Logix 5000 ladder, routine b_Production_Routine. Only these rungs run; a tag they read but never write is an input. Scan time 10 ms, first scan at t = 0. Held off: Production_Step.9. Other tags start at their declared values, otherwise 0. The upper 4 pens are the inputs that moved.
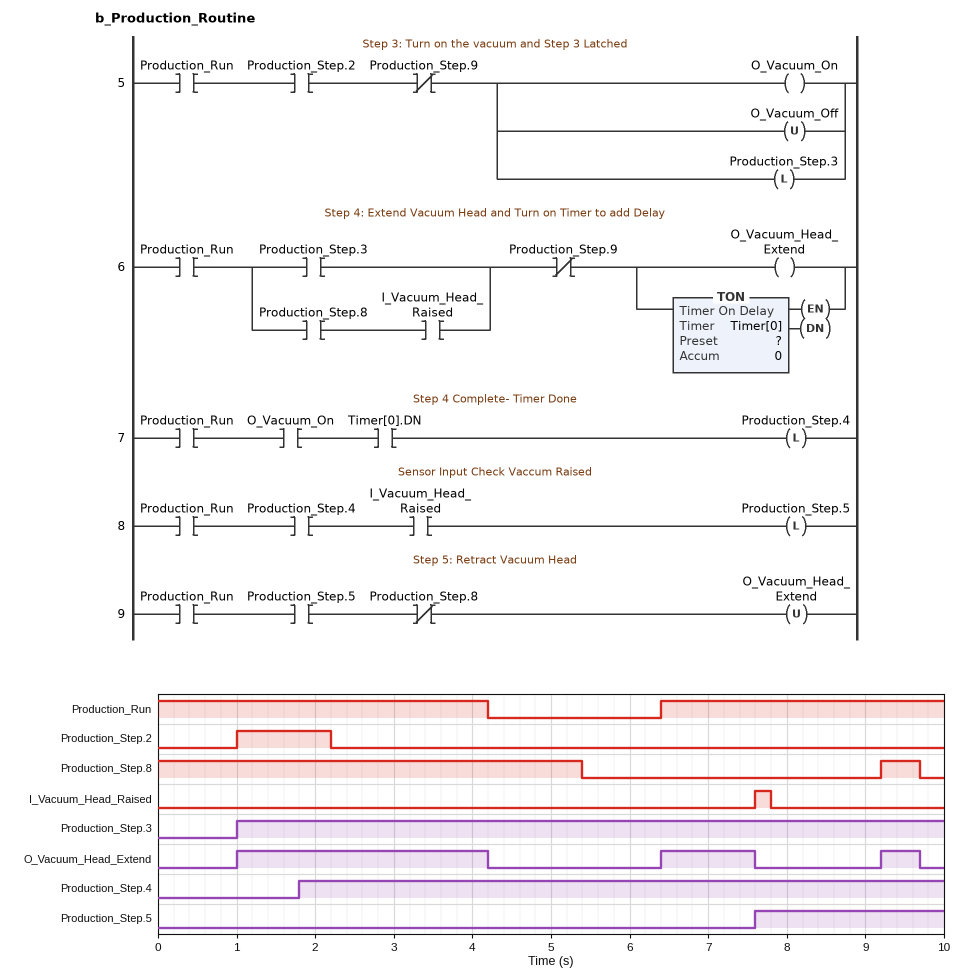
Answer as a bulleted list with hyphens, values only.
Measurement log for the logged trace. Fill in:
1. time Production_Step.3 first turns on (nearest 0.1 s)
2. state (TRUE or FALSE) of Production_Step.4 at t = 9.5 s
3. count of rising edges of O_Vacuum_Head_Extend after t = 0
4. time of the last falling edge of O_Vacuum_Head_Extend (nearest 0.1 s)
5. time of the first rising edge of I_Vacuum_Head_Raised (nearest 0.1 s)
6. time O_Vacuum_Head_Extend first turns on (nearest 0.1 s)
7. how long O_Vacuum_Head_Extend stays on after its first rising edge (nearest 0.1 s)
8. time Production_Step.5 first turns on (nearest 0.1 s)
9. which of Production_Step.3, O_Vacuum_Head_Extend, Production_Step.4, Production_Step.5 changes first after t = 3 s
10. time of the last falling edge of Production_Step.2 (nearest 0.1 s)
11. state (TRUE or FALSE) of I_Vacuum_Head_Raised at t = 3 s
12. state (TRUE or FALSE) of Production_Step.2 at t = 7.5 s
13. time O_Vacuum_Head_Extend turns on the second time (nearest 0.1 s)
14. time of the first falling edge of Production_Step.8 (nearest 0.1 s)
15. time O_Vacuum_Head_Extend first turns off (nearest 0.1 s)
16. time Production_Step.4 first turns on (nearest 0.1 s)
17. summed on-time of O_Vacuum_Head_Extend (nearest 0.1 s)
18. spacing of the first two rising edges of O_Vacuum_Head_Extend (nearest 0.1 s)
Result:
- 1.0 s
- TRUE
- 3
- 9.7 s
- 7.6 s
- 1.0 s
- 3.2 s
- 7.6 s
- O_Vacuum_Head_Extend
- 2.2 s
- FALSE
- FALSE
- 6.4 s
- 5.4 s
- 4.2 s
- 1.8 s
- 4.9 s
- 5.4 s
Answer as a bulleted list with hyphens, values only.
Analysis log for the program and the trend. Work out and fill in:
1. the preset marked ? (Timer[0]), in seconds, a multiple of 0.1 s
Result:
- 0.8 s
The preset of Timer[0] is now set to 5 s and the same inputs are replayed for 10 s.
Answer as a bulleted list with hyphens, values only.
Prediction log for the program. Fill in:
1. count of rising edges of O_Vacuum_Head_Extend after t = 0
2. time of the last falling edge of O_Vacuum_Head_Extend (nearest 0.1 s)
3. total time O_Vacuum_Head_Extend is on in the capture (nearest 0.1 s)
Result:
- 2
- 4.2 s
- 6.8 s
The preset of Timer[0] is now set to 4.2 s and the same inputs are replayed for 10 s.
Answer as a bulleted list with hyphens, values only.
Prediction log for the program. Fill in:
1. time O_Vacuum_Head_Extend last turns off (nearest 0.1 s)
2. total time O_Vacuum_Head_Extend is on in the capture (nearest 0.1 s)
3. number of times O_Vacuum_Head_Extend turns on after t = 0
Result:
- 4.2 s
- 6.8 s
- 2
